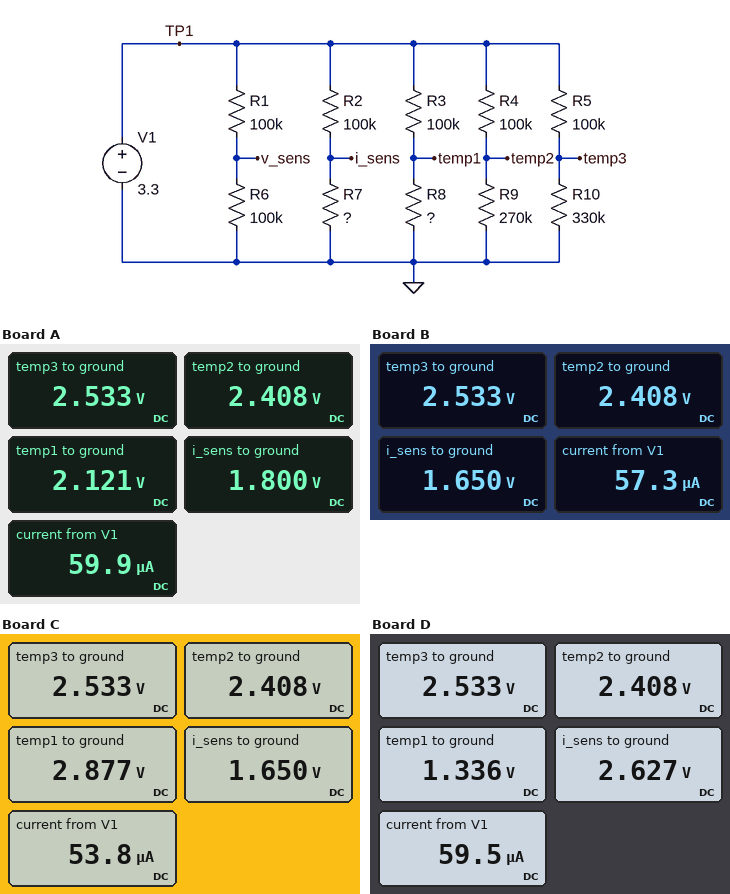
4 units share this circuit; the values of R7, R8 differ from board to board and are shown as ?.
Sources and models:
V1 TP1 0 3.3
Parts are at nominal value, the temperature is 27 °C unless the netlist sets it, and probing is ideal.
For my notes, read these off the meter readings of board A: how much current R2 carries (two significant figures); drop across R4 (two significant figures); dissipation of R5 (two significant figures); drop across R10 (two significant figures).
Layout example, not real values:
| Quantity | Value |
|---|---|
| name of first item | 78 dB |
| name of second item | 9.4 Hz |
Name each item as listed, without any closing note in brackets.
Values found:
| Quantity | Value |
|---|---|
| how much current R2 carries | 15 µA |
| drop across R4 | 890 mV |
| dissipation of R5 | 5.9 µW |
| drop across R10 | 2.5 V |
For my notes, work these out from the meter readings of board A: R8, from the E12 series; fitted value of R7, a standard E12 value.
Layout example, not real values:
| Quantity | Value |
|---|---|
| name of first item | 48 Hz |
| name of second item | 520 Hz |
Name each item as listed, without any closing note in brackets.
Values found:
| Quantity | Value |
|---|---|
| R8, from the E12 series | 180 kΩ |
| fitted value of R7, a standard E12 value | 120 kΩ |
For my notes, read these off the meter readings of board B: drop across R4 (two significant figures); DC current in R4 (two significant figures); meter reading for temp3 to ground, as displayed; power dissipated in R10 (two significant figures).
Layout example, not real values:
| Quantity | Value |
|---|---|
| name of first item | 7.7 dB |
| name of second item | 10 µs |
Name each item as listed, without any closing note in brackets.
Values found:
| Quantity | Value |
|---|---|
| drop across R4 | 890 mV |
| DC current in R4 | 8.9 µA |
| meter reading for temp3 to ground, as displayed | 2.533 V |
| power dissipated in R10 | 19 µW |
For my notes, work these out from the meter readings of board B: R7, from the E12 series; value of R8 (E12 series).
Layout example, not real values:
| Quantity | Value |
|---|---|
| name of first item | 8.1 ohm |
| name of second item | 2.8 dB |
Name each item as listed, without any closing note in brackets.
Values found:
| Quantity | Value |
|---|---|
| R7, from the E12 series | 100 kΩ |
| value of R8 | 330 kΩ |
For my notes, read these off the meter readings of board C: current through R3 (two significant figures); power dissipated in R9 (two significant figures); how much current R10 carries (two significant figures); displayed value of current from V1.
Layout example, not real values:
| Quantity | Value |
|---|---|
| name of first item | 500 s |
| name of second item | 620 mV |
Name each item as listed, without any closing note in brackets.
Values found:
| Quantity | Value |
|---|---|
| current through R3 | 4.2 µA |
| power dissipated in R9 | 21 µW |
| how much current R10 carries | 7.7 µA |
| displayed value of current from V1 | 53.8 µA |
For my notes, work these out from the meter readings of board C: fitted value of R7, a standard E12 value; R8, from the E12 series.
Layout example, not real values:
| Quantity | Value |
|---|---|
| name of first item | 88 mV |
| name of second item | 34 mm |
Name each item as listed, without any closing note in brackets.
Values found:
| Quantity | Value |
|---|---|
| fitted value of R7, a standard E12 value | 100 kΩ |
| R8, from the E12 series | 680 kΩ |
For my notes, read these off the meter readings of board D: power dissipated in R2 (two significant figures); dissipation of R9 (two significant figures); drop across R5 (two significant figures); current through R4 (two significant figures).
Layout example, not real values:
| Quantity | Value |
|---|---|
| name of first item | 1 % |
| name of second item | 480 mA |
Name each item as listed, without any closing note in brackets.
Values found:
| Quantity | Value |
|---|---|
| power dissipated in R2 | 4.5 µW |
| dissipation of R9 | 21 µW |
| drop across R5 | 770 mV |
| current through R4 | 8.9 µA |
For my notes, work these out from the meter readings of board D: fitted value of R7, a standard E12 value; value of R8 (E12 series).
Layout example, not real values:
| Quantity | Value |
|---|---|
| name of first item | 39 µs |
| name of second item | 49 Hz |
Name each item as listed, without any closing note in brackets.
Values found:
| Quantity | Value |
|---|---|
| fitted value of R7, a standard E12 value | 390 kΩ |
| value of R8 | 68 kΩ |
